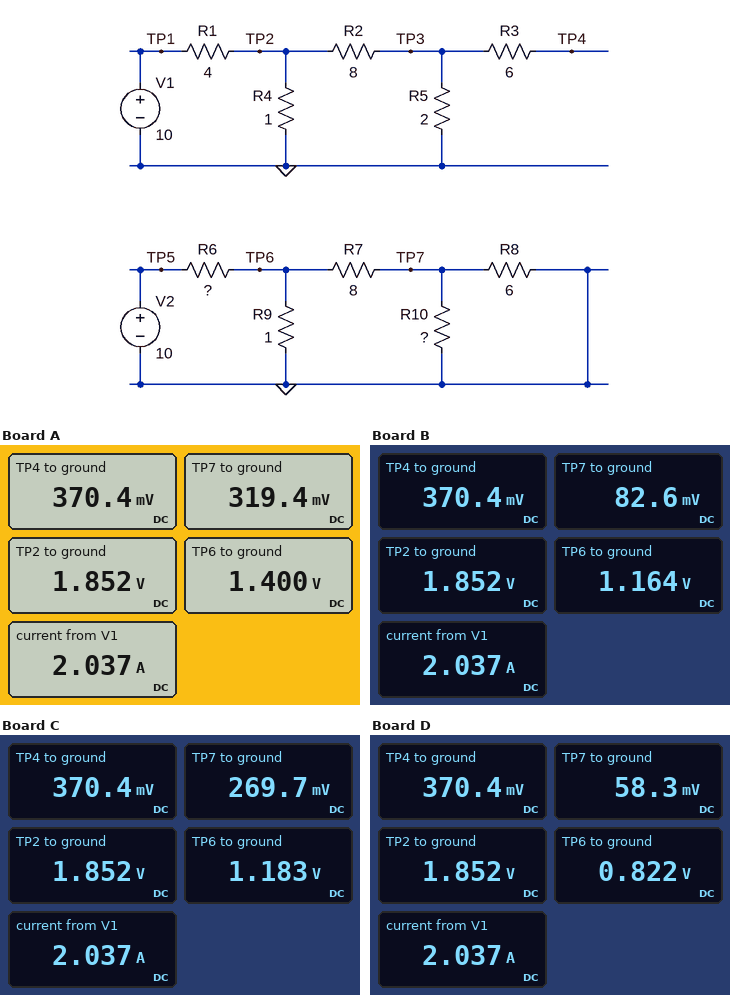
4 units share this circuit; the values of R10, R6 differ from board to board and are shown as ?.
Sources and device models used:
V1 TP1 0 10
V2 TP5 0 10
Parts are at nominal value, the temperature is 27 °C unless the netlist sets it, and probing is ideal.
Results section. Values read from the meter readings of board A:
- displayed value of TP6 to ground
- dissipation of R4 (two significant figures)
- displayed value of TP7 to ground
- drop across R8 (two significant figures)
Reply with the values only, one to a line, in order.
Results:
1.400 V
3.4 W
319.4 mV
320 mV
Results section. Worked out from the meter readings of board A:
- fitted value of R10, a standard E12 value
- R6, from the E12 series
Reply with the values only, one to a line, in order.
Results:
3.9 Ω
5.6 Ω
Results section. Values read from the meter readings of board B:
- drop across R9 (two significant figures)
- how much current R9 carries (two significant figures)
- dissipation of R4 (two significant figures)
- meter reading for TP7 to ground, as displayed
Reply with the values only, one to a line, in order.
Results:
1.2 V
1.2 A
3.4 W
82.6 mV
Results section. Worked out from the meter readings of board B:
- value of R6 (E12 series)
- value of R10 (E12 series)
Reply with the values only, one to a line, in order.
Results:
6.8 Ω
0.68 Ω
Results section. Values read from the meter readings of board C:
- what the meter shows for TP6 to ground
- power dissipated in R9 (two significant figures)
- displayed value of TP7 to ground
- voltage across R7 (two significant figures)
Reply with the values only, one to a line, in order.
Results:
1.183 V
1.4 W
269.7 mV
910 mV
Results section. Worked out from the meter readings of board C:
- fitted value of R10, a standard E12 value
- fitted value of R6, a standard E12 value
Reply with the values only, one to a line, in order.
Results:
3.9 Ω
6.8 Ω
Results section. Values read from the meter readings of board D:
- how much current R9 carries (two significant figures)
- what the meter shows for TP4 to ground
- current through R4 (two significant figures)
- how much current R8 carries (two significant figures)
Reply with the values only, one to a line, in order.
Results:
820 mA
370.4 mV
1.9 A
9.7 mA
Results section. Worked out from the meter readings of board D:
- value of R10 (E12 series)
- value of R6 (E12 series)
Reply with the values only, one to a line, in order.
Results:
0.68 Ω
10 Ω
